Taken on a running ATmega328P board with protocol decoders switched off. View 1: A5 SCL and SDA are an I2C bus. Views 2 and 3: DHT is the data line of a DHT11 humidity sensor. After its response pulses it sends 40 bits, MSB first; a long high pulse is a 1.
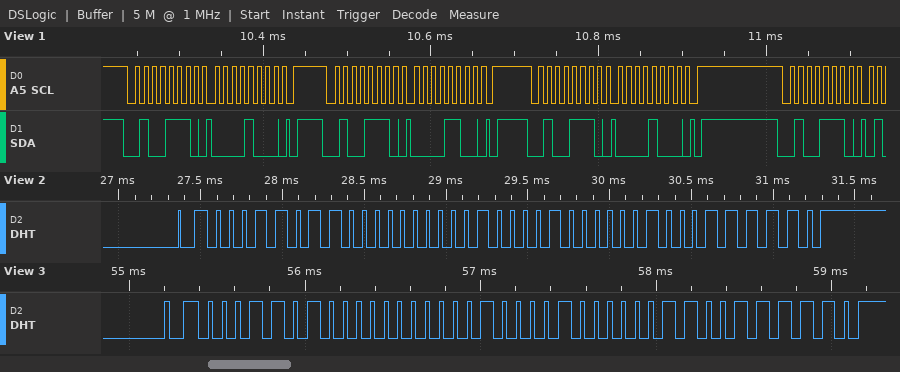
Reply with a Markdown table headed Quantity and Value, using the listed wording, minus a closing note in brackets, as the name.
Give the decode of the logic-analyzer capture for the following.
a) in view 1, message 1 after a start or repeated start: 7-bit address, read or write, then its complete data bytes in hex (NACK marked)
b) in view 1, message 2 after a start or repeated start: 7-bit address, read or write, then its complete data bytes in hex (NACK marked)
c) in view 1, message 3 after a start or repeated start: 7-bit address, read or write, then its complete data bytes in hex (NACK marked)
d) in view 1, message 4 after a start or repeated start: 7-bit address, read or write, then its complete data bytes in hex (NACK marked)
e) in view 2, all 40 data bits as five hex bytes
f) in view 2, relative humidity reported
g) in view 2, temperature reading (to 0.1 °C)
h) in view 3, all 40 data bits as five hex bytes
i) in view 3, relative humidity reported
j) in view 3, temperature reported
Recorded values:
| Quantity | Value |
|---|---|
| in view 1, message 1 after a start or repeated start: 7-bit address, read or write, then its complete data bytes in hex | 0x27 write: 08 |
| in view 1, message 2 after a start or repeated start: 7-bit address, read or write, then its complete data bytes in hex | 0x27 write: 0C |
| in view 1, message 3 after a start or repeated start: 7-bit address, read or write, then its complete data bytes in hex | 0x27 write: 08 |
| in view 1, message 4 after a start or repeated start: 7-bit address, read or write, then its complete data bytes in hex | 0x27 write |
| in view 2, all 40 data bits as five hex bytes | 1B 00 21 02 3E |
| in view 2, relative humidity reported | 27 % |
| in view 2, temperature reading | 33.2 °C |
| in view 3, all 40 data bits as five hex bytes | 1A 00 21 03 3E |
| in view 3, relative humidity reported | 26 % |
| in view 3, temperature reported | 33.3 °C |
